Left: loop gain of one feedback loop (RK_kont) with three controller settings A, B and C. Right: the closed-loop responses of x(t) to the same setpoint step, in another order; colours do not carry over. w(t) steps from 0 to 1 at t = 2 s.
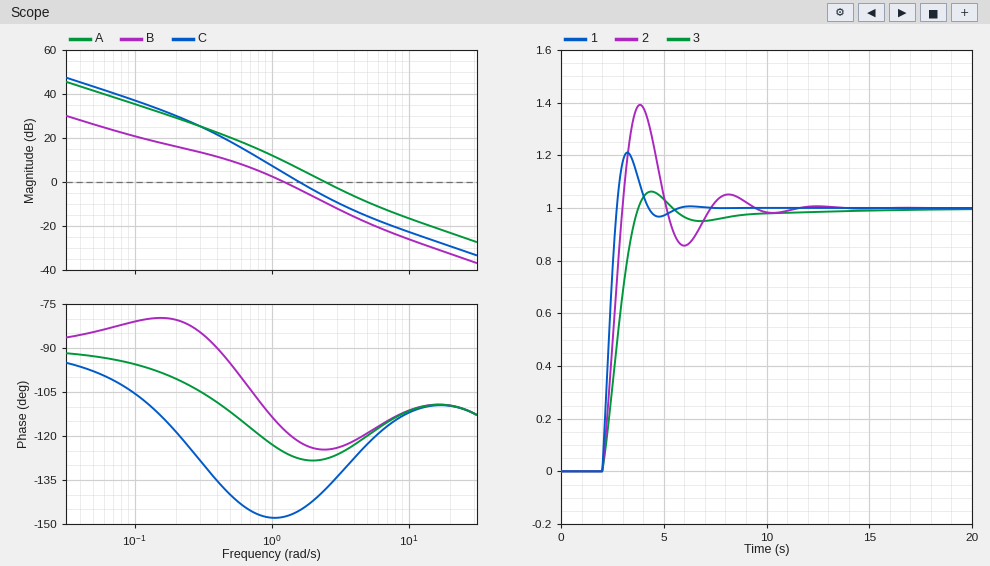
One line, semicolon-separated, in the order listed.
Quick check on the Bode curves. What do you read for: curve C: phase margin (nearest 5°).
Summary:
35°
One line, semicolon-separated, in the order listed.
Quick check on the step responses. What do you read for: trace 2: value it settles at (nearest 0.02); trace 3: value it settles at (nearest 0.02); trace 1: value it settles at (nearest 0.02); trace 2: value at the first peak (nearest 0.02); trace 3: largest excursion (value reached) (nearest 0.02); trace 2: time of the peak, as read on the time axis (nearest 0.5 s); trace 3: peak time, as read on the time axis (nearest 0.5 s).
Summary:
1.00; 1.00; 1.00; 1.40; 1.06; 4.0 s; 4.5 s
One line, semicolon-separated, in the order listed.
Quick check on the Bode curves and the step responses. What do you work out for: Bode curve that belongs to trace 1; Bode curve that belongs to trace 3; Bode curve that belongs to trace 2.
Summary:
A; B; C
